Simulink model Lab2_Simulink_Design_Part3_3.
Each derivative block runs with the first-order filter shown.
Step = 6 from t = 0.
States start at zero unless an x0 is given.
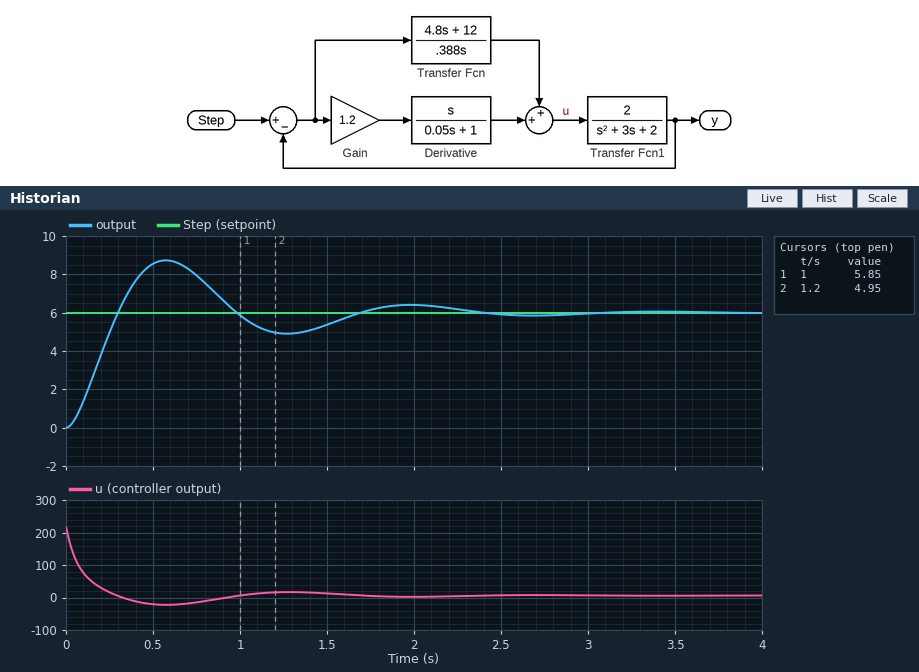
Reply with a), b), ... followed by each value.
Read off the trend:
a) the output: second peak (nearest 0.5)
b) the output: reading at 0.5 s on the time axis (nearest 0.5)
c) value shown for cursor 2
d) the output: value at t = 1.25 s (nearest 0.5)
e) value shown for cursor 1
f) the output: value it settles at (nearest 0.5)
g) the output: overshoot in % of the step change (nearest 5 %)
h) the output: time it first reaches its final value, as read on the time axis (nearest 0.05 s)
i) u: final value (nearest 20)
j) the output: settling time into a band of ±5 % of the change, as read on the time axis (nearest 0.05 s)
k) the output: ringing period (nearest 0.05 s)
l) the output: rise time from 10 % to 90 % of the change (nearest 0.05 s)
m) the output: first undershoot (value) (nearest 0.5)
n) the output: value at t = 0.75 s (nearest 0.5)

a) 6.5
b) 8.5
c) 4.95
d) 5.0
e) 5.85
f) 6.0
g) 45 %
h) 0.30 s
i) 0
j) 2.15 s
k) 1.40 s
l) 0.20 s
m) 5.0
n) 8.0
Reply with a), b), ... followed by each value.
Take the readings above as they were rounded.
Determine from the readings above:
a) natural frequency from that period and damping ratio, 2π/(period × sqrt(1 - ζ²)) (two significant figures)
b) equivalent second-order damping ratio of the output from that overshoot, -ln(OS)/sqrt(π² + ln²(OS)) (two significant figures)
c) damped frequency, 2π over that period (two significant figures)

a) 4.6 rad/s
b) 0.25
c) 4.5 rad/s
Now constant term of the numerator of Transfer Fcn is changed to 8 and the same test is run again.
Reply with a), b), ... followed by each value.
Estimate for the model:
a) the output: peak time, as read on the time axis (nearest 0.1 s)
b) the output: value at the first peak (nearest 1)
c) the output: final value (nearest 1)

a) 0.6 s
b) 8
c) 6
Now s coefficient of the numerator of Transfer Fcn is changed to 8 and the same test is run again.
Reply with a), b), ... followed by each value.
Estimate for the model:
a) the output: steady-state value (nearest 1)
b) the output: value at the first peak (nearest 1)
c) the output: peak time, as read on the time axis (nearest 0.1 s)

a) 6
b) 9
c) 0.4 s
